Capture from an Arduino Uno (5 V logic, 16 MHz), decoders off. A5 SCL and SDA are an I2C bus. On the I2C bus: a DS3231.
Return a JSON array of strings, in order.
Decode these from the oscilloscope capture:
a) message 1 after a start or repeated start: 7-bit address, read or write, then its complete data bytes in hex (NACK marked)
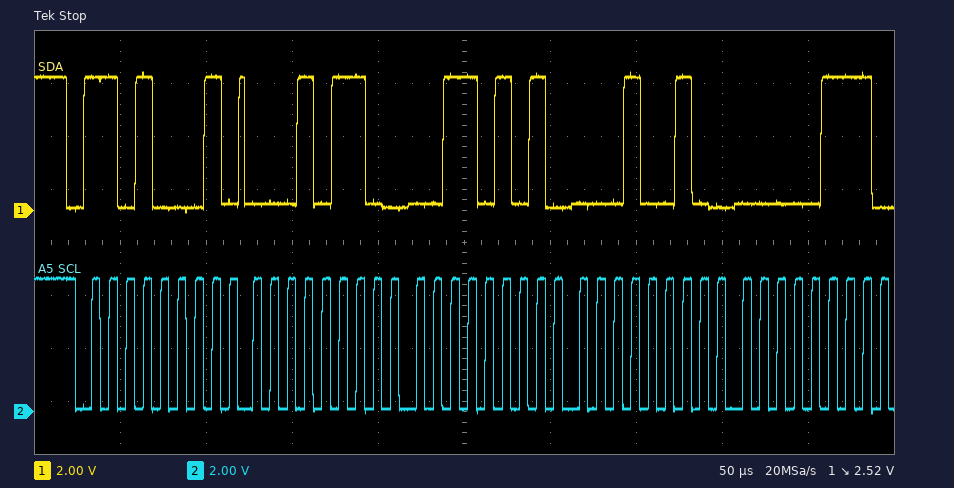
["0x68 read: 16 35 12 07"]
